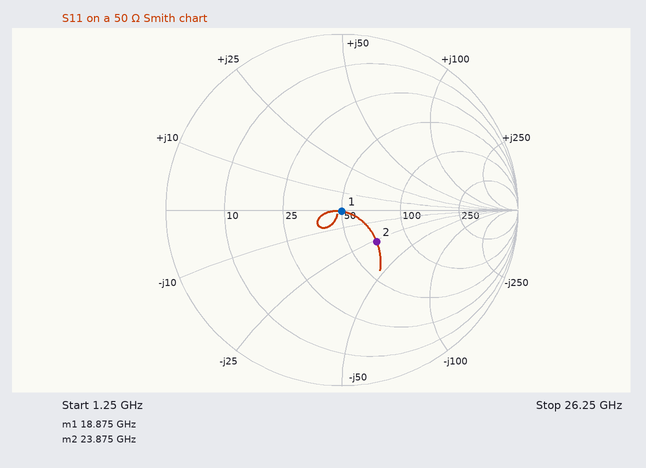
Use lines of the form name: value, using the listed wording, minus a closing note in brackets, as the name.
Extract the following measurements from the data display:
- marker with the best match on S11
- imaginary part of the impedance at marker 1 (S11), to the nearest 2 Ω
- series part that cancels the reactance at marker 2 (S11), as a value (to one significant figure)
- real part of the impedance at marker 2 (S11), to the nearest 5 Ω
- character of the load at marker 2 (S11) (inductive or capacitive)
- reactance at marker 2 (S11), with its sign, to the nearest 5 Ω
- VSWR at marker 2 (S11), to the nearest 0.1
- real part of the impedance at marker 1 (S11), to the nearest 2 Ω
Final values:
marker with the best match on S11: marker 1
imaginary part of the impedance at marker 1 (S11), to the nearest 2 Ω: 0 Ω
series part that cancels the reactance at marker 2 (S11), as a value: 200 pH
real part of the impedance at marker 2 (S11), to the nearest 5 Ω: 70 Ω
character of the load at marker 2 (S11): capacitive
reactance at marker 2 (S11), with its sign, to the nearest 5 Ω: -25 Ω
VSWR at marker 2 (S11), to the nearest 0.1: 1.7
real part of the impedance at marker 1 (S11), to the nearest 2 Ω: 50 Ω
